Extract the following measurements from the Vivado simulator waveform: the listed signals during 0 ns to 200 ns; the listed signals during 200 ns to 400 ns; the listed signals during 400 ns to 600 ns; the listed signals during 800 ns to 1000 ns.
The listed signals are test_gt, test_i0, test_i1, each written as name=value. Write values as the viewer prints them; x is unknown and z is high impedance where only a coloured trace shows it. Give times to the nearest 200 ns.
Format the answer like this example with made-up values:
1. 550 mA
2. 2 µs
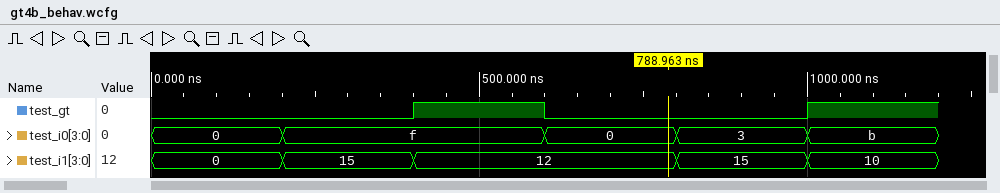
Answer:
1. test_gt=0, test_i0=0, test_i1=0
2. test_gt=0, test_i0=f, test_i1=15
3. test_gt=1, test_i0=f, test_i1=12
4. test_gt=0, test_i0=3, test_i1=15
